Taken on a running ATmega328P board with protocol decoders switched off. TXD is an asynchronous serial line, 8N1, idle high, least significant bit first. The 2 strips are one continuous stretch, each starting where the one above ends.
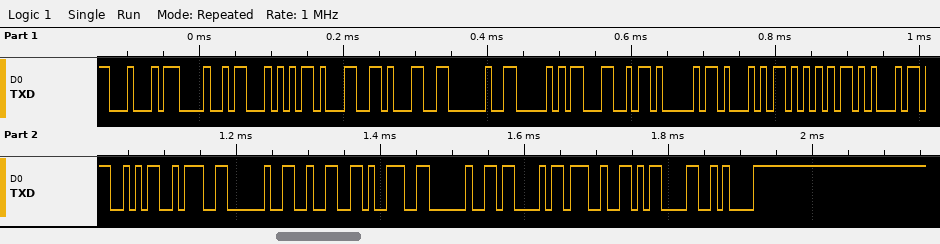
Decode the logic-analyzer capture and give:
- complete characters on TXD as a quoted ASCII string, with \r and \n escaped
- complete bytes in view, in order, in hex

"DHT11 PLAQUES: 29 C'\r\n"
44 48 54 31 31 20 50 4C 41 51 55 45 53 3A 20 32 39 20 43 27 0D 0A
